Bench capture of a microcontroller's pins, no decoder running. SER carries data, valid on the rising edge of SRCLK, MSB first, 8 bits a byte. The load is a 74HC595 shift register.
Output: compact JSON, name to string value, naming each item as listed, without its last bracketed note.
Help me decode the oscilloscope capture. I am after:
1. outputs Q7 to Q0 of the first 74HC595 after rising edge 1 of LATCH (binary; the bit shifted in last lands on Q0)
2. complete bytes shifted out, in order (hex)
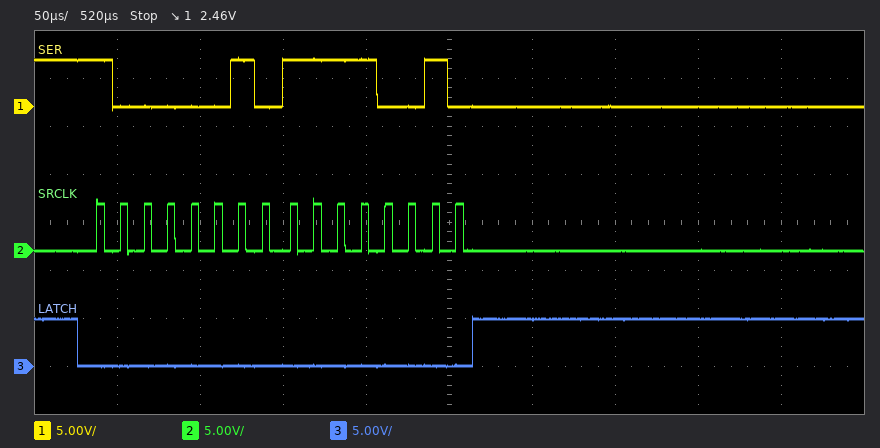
{"outputs Q7 to Q0 of the first 74HC595 after rising edge 1 of LATCH": "11110010", "complete bytes shifted out, in order": "0x82 0xF2"}
